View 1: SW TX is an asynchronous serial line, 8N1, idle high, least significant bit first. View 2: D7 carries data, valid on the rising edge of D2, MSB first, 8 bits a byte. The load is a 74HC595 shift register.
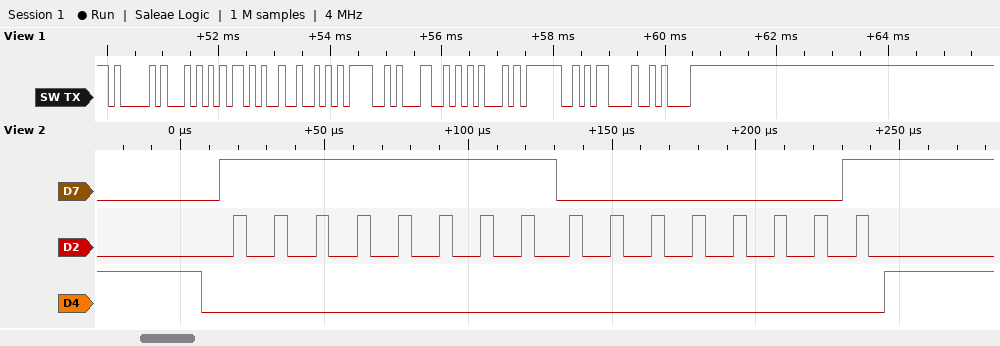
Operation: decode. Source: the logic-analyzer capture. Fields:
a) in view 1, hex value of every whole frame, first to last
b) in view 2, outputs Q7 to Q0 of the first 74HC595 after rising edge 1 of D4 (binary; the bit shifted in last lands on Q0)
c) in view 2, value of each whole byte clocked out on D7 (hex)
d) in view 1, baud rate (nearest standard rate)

0x41 0x54 0x2B 0x52 0x4F 0x4C 0x45 0x3F 0x0D 0x0A
00000001
0xFF 0x01
9600 baud
